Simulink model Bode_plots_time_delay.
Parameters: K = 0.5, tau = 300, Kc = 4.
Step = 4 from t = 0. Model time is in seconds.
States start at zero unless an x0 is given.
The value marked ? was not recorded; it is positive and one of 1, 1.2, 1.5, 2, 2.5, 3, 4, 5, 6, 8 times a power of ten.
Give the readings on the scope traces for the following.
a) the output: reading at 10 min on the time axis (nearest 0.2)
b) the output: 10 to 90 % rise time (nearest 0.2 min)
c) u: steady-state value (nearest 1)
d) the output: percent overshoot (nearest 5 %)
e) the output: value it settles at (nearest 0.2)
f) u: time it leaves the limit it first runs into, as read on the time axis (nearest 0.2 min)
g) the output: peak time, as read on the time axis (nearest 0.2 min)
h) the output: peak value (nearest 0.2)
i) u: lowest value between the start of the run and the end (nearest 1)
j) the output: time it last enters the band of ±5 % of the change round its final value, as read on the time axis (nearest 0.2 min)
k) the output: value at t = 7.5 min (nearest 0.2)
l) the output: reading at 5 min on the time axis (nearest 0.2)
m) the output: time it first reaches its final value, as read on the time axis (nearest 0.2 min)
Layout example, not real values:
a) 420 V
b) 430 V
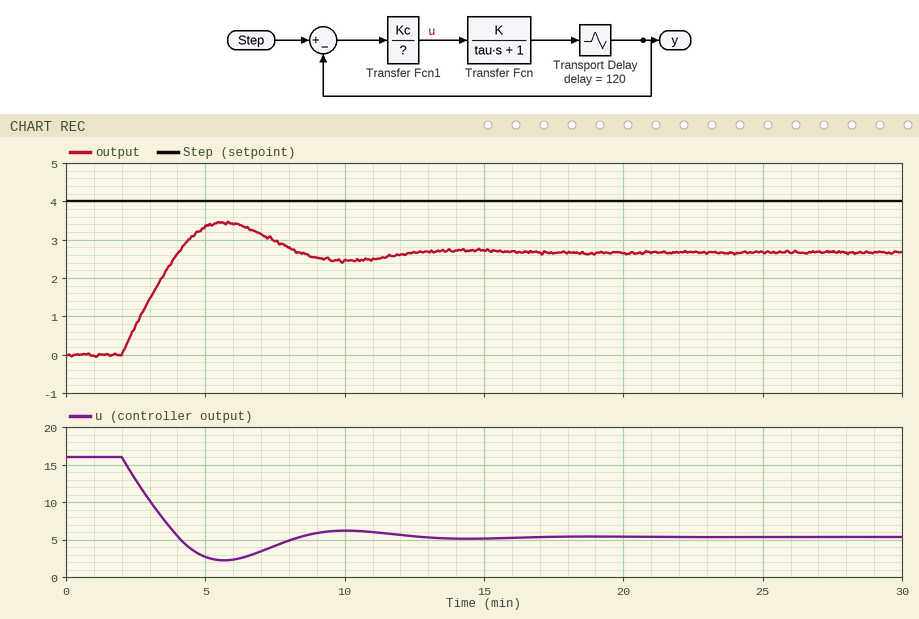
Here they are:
a) 2.4
b) 1.6 min
c) 5
d) 30 %
e) 2.6
f) 2.0 min
g) 5.6 min
h) 3.4
i) 2
j) 11.4 min
k) 3.0
l) 3.4
m) 4.0 min
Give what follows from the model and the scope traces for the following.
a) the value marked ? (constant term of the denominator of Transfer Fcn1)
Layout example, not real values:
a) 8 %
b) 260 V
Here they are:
a) 1
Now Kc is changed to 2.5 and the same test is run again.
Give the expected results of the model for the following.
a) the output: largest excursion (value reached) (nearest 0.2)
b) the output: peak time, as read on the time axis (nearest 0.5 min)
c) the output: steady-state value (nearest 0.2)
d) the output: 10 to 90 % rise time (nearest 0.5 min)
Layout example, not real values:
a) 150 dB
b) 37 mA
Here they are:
a) 2.4
b) 7.0 min
c) 2.2
d) 2.5 min
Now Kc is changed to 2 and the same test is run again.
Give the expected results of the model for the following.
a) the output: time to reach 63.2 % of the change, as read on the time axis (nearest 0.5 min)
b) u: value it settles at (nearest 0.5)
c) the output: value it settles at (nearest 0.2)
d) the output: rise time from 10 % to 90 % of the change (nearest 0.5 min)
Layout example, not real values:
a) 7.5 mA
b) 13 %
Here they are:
a) 4.0 min
b) 4.0
c) 2.0
d) 3.0 min
